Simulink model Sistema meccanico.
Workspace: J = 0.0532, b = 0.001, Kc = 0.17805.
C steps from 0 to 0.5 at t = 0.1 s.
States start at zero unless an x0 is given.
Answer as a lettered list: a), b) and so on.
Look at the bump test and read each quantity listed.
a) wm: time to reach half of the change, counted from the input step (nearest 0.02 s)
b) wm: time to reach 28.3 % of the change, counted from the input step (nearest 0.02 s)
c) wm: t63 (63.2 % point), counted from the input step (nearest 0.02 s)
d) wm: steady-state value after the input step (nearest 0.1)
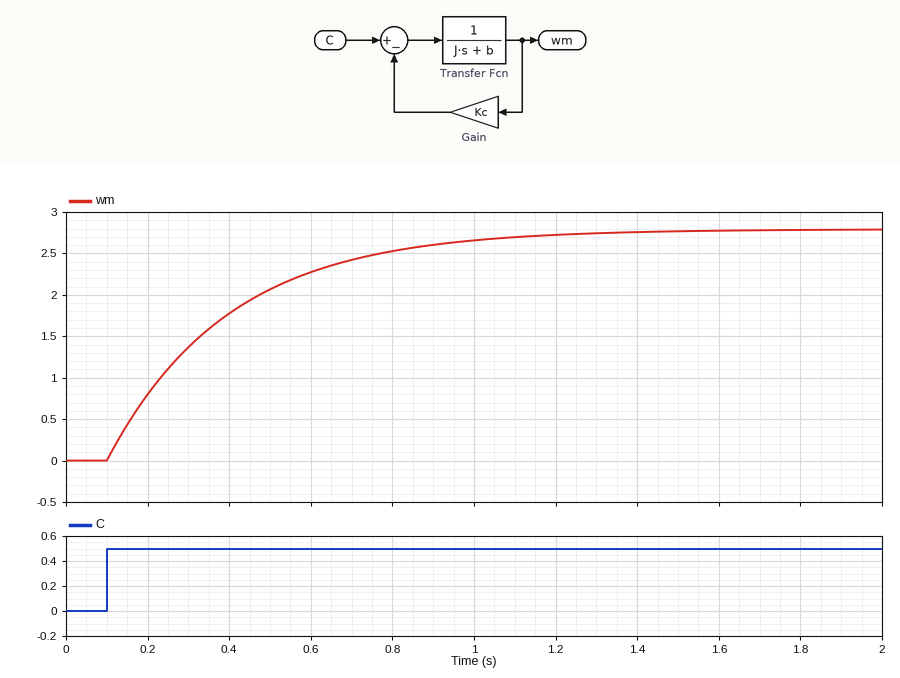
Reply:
a) 0.20 s
b) 0.10 s
c) 0.30 s
d) 2.8
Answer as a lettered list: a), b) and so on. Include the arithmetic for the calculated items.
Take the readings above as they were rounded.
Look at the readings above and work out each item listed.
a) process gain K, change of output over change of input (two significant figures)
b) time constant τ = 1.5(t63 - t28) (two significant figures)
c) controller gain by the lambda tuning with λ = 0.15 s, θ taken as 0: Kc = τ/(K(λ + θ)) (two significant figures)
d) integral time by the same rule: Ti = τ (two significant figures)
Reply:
a) (2.8 - 0) / 0.5 = 5.6
b) 1.5 × (0.3 - 0.1) = 0.30 s
c) 0.3 / (5.6 × (0.15 + 0)) = 0.36
d) 0.30 s
